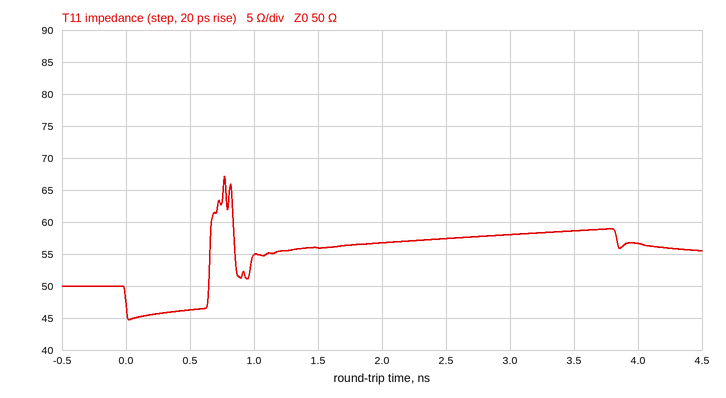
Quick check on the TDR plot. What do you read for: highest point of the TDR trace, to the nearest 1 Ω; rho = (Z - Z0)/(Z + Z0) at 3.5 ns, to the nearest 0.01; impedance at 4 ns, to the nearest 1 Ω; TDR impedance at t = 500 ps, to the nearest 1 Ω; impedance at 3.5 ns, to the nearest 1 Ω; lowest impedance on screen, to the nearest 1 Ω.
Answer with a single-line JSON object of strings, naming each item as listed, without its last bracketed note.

{"highest point of the TDR trace, to the nearest 1 Ω": "67 Ω", "rho = (Z - Z0)/(Z + Z0) at 3.5 ns, to the nearest 0.01": "+0.08", "impedance at 4 ns, to the nearest 1 Ω": "57 Ω", "TDR impedance at t = 500 ps, to the nearest 1 Ω": "46 Ω", "impedance at 3.5 ns, to the nearest 1 Ω": "59 Ω", "lowest impedance on screen, to the nearest 1 Ω": "45 Ω"}
